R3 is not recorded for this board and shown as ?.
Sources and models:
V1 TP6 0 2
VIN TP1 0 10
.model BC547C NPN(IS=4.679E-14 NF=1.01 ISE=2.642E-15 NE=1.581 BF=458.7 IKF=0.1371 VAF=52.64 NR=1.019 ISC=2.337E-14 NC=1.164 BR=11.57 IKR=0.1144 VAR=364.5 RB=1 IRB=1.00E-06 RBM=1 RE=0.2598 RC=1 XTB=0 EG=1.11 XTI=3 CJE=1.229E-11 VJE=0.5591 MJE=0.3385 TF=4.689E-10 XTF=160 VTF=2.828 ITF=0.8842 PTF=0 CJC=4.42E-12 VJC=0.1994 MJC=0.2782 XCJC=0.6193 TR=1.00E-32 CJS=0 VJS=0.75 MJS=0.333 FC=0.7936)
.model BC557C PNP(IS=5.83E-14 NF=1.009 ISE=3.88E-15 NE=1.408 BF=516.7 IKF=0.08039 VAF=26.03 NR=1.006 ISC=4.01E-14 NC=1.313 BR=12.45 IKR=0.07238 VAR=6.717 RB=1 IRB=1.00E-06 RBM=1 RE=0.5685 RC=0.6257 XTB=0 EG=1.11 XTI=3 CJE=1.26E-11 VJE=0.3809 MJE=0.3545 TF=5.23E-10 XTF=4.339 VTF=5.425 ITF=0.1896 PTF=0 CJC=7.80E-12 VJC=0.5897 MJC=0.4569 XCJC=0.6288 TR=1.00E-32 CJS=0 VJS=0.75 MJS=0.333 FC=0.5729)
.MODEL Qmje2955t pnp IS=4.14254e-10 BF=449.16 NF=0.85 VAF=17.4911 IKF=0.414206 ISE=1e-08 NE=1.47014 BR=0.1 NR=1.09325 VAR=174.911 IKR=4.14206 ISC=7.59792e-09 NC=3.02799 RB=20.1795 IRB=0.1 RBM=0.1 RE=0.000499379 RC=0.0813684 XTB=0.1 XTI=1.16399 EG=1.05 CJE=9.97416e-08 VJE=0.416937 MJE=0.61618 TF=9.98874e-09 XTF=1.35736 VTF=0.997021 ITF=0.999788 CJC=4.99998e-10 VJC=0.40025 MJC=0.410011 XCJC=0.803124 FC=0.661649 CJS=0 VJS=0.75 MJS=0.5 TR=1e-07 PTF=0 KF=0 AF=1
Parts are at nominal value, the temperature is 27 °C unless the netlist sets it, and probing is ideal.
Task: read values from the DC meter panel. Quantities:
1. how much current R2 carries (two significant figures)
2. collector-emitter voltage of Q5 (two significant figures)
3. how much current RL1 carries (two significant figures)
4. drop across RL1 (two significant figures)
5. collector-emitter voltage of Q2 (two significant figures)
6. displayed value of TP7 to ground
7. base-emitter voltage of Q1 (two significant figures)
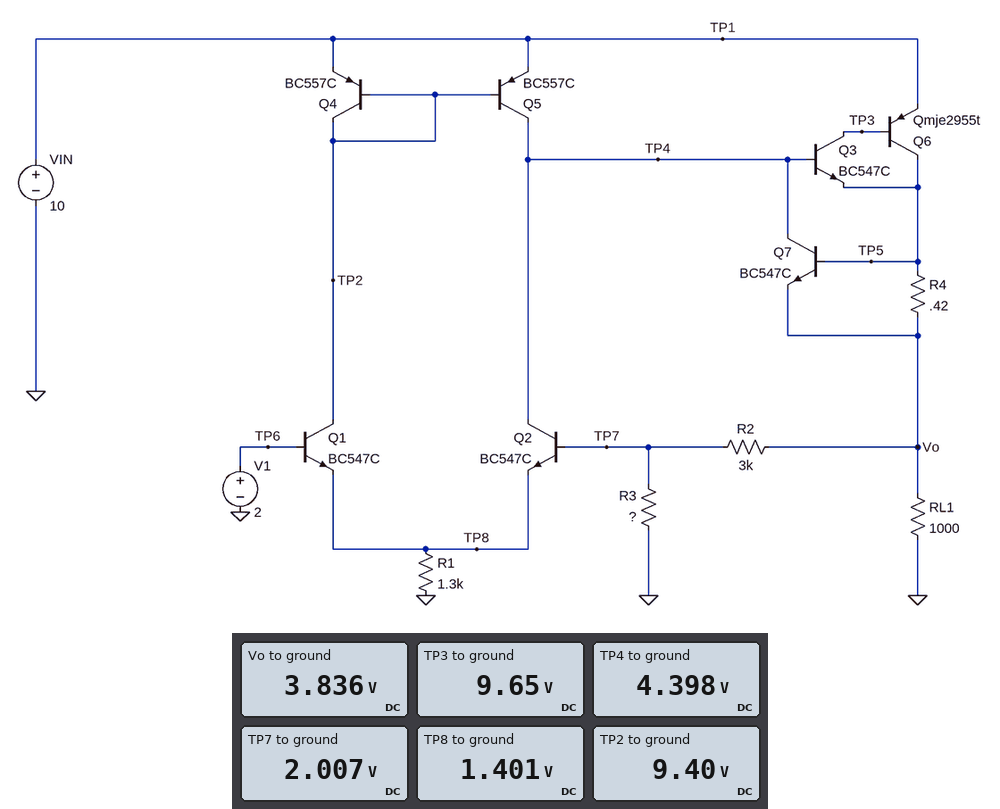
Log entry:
610 µA
-5.6 V
3.8 mA
3.8 V
3.0 V
2.007 V
600 mV
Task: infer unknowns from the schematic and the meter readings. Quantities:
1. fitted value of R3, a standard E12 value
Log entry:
3.3 kΩ
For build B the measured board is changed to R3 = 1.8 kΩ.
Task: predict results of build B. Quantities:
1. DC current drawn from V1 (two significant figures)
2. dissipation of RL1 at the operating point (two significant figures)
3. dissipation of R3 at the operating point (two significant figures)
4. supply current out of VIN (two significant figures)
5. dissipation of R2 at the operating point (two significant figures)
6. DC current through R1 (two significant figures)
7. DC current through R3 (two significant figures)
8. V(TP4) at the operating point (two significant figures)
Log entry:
970 nA
29 mW
2.2 mW
7.5 mA
3.7 mW
1.1 mA
1.1 mA
5.9 V
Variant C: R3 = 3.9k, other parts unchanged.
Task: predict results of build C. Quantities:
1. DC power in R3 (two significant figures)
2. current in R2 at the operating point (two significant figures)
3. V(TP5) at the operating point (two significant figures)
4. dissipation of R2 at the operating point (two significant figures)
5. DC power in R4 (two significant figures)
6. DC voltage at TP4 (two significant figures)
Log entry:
1.0 mW
520 µA
3.6 V
800 µW
7.0 µW
4.1 V
